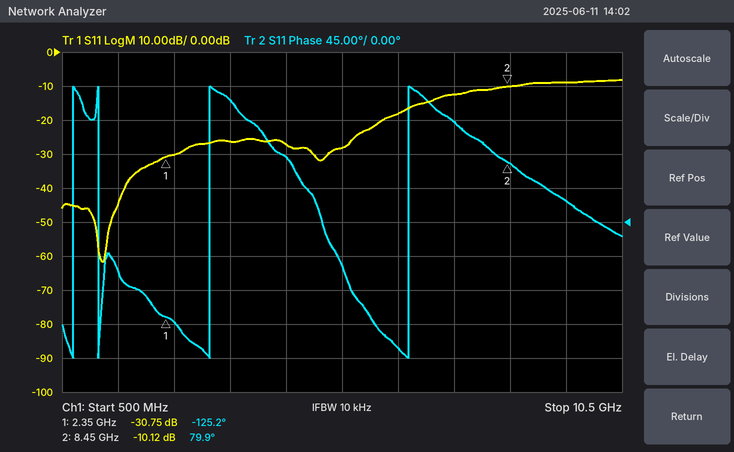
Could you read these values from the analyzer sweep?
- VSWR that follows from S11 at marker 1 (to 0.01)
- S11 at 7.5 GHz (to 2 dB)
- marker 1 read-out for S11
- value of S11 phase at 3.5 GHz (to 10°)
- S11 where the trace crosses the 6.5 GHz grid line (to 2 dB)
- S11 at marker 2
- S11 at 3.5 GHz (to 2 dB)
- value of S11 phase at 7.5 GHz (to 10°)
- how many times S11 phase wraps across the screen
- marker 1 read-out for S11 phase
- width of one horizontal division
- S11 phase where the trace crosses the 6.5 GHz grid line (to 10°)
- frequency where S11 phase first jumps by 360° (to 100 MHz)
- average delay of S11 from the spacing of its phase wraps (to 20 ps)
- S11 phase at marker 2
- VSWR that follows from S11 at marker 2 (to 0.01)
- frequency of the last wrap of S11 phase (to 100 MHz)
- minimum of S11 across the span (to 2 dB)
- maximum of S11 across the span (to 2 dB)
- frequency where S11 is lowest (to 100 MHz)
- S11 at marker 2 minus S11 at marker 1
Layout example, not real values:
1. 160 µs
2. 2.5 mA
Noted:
1. 1.06
2. -12 dB
3. -30.75 dB
4. 160°
5. -18 dB
6. -10.12 dB
7. -26 dB
8. 130°
9. 4
10. -125.2°
11. 1 GHz
12. -170°
13. 700 MHz
14. 500 ps
15. 79.9°
16. 1.91
17. 6.7 GHz
18. -62 dB
19. -8 dB
20. 1.2 GHz
21. 20.63 dB
